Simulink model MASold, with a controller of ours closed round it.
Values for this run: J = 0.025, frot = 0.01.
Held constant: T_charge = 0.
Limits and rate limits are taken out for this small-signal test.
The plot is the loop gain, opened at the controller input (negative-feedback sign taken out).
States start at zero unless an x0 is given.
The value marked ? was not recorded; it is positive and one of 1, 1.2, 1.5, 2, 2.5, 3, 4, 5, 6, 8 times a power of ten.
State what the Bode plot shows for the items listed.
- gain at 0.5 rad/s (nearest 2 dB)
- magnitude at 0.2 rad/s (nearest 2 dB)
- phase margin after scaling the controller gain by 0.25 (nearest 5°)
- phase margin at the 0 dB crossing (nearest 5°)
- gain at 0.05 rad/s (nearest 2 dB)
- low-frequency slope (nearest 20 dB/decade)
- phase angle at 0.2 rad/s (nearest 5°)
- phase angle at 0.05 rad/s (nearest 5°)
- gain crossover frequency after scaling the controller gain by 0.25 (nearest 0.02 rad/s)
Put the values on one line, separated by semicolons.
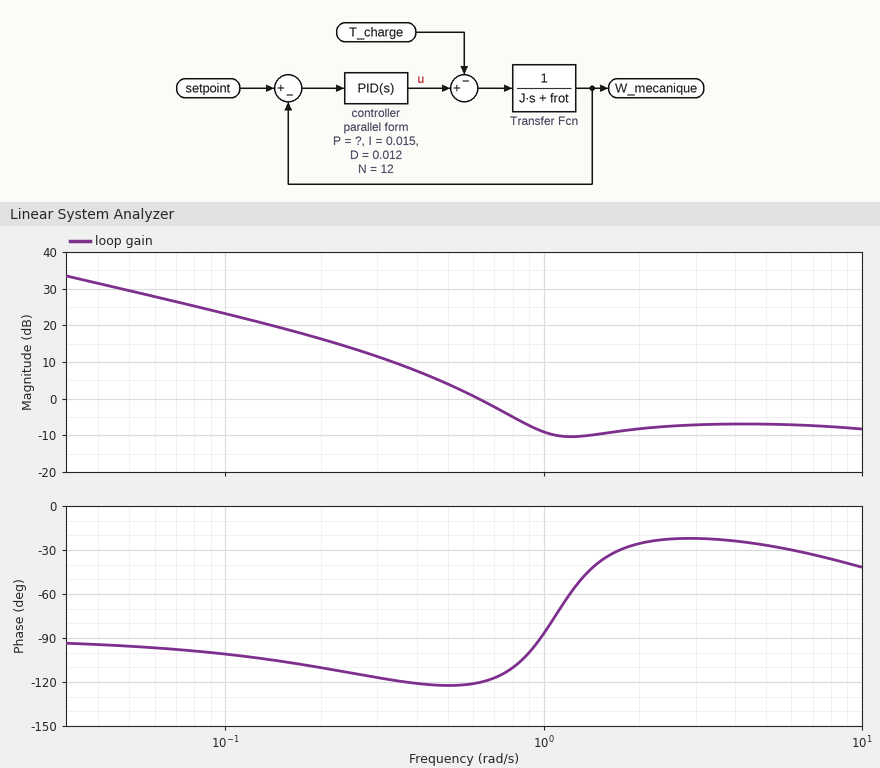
4 dB; 16 dB; 65°; 60°; 30 dB; -20 dB/decade; -110°; -95°; 0.28 rad/s
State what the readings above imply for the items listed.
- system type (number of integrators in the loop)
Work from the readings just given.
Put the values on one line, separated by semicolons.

1
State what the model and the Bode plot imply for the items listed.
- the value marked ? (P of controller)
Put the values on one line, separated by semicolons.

0.008
